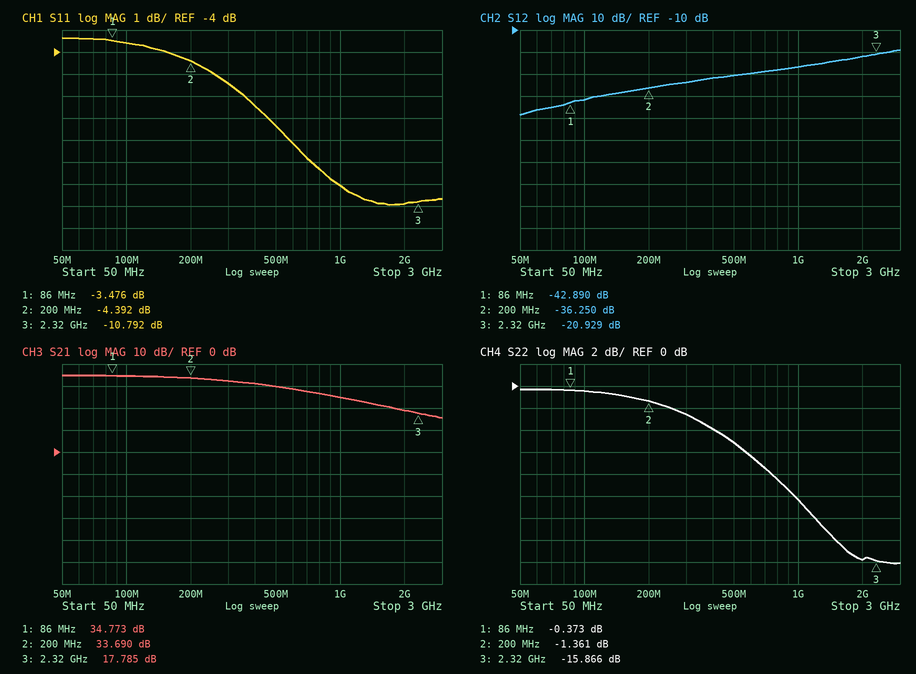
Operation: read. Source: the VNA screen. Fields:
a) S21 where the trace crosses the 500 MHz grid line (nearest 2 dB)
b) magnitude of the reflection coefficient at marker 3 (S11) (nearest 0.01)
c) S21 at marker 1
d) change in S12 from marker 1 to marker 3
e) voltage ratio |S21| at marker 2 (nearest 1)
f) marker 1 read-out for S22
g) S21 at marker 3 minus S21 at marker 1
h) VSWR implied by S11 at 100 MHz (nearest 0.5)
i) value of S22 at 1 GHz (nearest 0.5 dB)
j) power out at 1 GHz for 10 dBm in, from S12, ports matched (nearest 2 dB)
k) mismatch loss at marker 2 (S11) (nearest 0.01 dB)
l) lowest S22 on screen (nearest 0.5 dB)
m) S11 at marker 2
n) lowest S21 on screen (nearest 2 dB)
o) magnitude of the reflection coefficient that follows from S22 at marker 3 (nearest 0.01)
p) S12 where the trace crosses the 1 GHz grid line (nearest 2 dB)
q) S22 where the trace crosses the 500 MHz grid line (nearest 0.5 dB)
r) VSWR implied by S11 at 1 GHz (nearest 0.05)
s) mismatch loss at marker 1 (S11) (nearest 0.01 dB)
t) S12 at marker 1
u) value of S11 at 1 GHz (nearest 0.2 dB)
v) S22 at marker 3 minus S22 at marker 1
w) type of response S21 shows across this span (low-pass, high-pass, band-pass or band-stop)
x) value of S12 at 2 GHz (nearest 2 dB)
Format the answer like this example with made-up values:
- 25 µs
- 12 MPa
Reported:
- 30 dB
- 0.29
- 34.773 dB
- 21.961 dB
- 48
- -0.373 dB
- -16.988 dB
- 5.0
- -10.5 dB
- -16 dBm
- 1.96 dB
- -16.0 dB
- -4.392 dB
- 16 dB
- 0.16
- -26 dB
- -5.0 dB
- 1.90
- 2.59 dB
- -42.890 dB
- -10.0 dB
- -15.493 dB
- low-pass
- -22 dB
